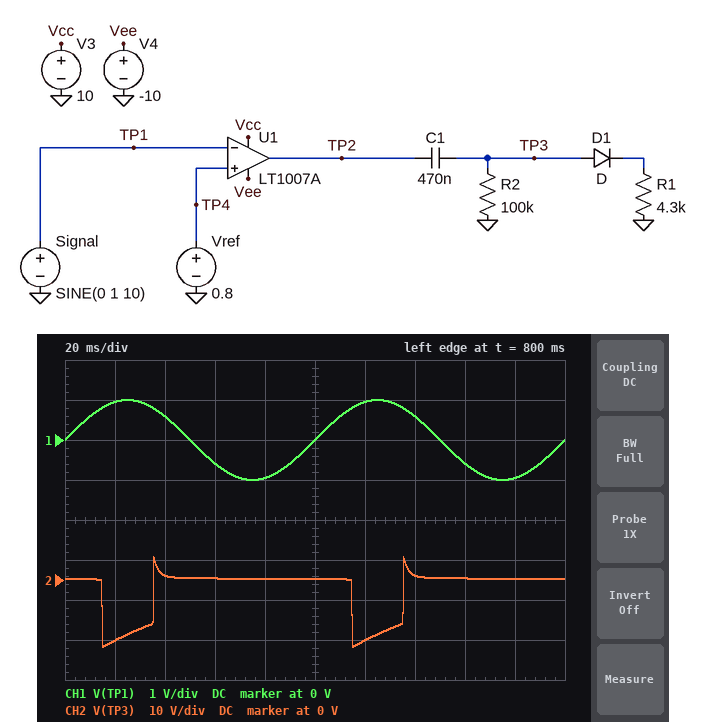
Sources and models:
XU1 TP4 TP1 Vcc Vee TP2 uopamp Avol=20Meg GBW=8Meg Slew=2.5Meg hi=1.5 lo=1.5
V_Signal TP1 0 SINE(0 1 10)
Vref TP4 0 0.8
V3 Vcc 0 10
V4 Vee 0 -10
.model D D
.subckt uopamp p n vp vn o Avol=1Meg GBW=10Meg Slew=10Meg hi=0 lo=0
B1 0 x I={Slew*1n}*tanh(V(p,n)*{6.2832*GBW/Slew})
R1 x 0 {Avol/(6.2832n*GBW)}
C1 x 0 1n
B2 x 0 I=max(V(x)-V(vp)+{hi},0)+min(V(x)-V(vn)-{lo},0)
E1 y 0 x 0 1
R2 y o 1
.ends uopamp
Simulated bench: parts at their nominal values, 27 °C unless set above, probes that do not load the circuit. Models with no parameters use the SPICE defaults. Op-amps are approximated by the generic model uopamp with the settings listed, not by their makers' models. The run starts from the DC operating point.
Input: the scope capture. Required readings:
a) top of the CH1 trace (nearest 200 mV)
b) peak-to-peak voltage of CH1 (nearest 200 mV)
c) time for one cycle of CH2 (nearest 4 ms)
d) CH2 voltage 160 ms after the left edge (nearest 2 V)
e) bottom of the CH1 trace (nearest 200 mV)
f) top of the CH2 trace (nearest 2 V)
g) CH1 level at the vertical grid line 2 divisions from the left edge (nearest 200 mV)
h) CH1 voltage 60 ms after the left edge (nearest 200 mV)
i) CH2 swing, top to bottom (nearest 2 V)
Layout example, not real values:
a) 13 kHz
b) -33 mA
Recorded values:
a) 1.0 V
b) 2.0 V
c) 100 ms
d) 0 V
e) -1.0 V
f) 6 V
g) 600 mV
h) -600 mV
i) 22 V
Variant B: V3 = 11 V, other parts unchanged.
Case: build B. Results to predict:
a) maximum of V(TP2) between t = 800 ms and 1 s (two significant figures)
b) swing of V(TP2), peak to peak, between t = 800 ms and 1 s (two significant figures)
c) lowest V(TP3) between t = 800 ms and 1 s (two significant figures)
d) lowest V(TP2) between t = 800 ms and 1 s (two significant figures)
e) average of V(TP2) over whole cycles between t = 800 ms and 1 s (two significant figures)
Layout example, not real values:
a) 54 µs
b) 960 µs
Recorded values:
a) 9.5 V
b) 18 V
c) -18 V
d) -8.5 V
e) 5.8 V
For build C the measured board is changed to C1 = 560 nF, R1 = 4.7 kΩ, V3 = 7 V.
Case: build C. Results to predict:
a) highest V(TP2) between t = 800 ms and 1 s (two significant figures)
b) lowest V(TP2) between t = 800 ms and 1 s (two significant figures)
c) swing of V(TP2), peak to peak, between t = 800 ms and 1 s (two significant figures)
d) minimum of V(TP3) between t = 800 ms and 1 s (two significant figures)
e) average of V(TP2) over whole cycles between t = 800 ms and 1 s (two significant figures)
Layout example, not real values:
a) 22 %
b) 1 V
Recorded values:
a) 5.5 V
b) -8.5 V
c) 14 V
d) -14 V
e) 2.6 V
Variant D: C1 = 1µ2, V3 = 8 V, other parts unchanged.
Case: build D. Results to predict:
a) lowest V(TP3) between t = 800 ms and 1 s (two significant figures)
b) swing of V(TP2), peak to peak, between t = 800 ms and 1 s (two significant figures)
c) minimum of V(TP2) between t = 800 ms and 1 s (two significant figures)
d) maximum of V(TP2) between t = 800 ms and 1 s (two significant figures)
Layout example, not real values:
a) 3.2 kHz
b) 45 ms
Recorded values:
a) -15 V
b) 15 V
c) -8.5 V
d) 6.5 V
